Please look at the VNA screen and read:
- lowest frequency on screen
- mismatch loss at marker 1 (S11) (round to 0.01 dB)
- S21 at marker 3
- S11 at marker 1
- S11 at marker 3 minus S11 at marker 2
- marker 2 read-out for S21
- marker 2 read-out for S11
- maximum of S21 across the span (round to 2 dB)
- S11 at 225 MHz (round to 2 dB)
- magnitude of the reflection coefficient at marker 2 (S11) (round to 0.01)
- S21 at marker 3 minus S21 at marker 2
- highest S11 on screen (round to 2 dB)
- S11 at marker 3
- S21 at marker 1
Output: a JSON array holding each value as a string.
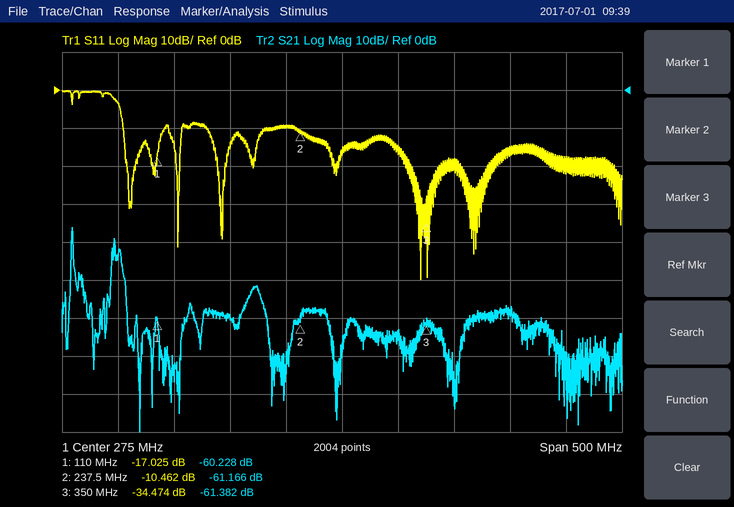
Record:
["25 MHz", "0.09 dB", "-61.382 dB", "-17.025 dB", "-24.012 dB", "-61.166 dB", "-10.462 dB", "-36 dB", "-10 dB", "0.30", "-0.216 dB", "0 dB", "-34.474 dB", "-60.228 dB"]
